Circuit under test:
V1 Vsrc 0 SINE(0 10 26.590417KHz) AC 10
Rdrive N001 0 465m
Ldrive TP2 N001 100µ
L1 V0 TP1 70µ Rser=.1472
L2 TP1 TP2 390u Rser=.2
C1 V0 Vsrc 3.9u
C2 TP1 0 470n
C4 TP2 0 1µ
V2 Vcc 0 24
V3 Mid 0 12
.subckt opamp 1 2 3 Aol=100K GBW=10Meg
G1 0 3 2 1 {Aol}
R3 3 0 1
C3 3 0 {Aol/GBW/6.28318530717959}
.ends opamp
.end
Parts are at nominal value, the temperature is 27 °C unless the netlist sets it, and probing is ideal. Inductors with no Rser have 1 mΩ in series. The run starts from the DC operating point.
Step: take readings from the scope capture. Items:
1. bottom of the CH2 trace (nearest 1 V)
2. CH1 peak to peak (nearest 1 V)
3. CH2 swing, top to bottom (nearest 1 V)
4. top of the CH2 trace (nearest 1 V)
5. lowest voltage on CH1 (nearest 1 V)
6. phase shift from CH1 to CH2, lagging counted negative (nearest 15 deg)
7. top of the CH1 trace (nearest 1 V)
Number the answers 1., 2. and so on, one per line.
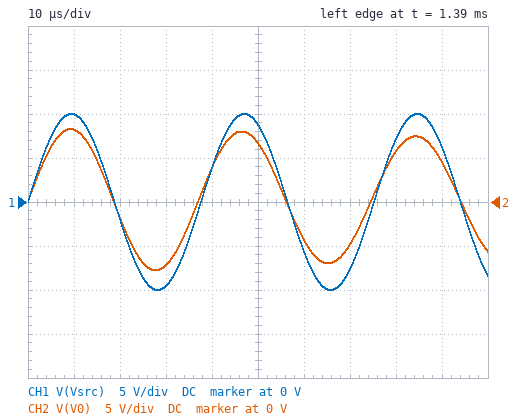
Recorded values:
1. -8 V
2. 20 V
3. 16 V
4. 8 V
5. -10 V
6. 0 deg
7. 10 V
